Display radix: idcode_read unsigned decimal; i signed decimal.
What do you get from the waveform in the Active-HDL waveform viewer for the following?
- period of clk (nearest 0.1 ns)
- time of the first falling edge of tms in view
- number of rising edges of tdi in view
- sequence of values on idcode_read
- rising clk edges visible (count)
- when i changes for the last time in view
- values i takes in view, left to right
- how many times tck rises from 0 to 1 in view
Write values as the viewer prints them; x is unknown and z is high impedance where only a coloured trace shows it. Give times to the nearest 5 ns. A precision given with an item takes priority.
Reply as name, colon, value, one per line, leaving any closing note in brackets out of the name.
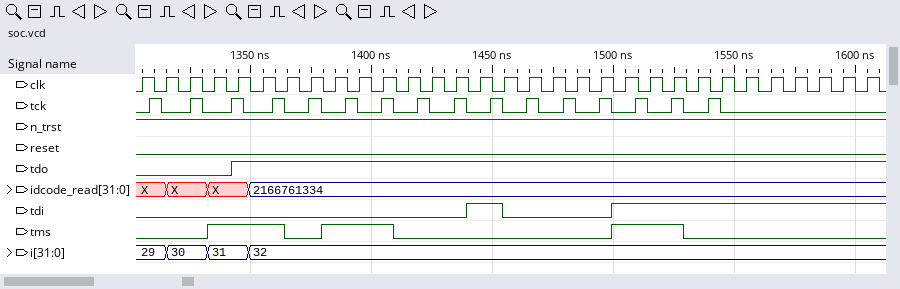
period of clk: 10 ns
time of the first falling edge of tms in view: 1365 ns
number of rising edges of tdi in view: 2
sequence of values on idcode_read: X, X, X, 2166761334
rising clk edges visible: 31
when i changes for the last time in view: 1350 ns
values i takes in view, left to right: 29, 30, 31, 32
how many times tck rises from 0 to 1 in view: 16
